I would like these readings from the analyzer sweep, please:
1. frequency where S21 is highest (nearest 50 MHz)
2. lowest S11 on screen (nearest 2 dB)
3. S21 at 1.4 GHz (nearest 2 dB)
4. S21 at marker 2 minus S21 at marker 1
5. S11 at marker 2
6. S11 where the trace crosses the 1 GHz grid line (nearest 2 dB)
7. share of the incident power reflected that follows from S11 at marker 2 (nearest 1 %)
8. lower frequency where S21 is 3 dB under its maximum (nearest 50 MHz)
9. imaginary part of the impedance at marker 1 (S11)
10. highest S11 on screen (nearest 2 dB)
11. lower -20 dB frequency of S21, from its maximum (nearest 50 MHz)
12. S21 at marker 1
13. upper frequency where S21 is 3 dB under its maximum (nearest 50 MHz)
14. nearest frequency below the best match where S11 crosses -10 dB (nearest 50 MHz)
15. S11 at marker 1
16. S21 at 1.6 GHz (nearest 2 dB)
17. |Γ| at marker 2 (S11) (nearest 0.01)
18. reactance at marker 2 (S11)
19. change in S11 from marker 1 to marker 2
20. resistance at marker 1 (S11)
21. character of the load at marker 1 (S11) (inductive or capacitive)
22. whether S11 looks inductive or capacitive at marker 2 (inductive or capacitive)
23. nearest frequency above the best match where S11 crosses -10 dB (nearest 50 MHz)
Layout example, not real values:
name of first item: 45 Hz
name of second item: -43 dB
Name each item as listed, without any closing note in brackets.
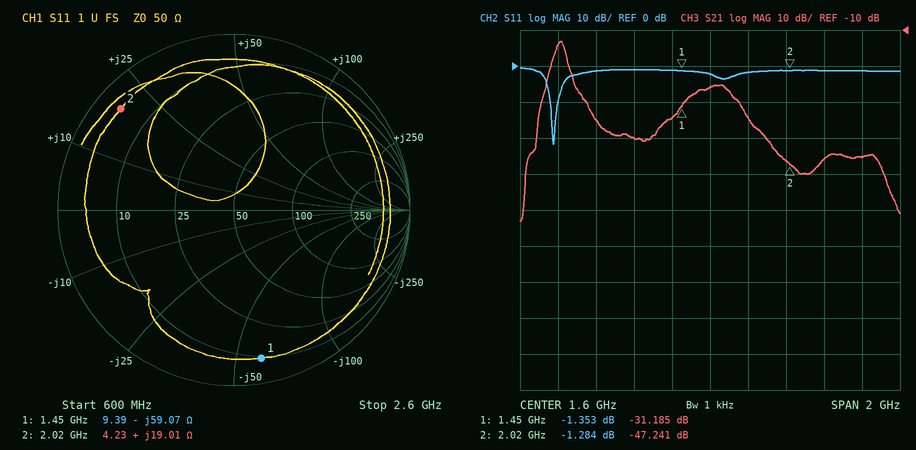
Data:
frequency where S21 is highest: 800 MHz
lowest S11 on screen: -22 dB
S21 at 1.4 GHz: -34 dB
S21 at marker 2 minus S21 at marker 1: -16.056 dB
S11 at marker 2: -1.284 dB
S11 where the trace crosses the 1 GHz grid line: -2 dB
share of the incident power reflected that follows from S11 at marker 2: 74 %
lower frequency where S21 is 3 dB under its maximum: 800 MHz
imaginary part of the impedance at marker 1: -59.07 Ω
highest S11 on screen: 0 dB
lower -20 dB frequency of S21, from its maximum: 700 MHz
S21 at marker 1: -31.185 dB
upper frequency where S21 is 3 dB under its maximum: 850 MHz
nearest frequency below the best match where S11 crosses -10 dB: 750 MHz
S11 at marker 1: -1.353 dB
S21 at 1.6 GHz: -26 dB
|Γ| at marker 2 (S11): 0.86
reactance at marker 2: +19.01 Ω
change in S11 from marker 1 to marker 2: 0.069 dB
resistance at marker 1: 9.39 Ω
character of the load at marker 1 (S11): capacitive
whether S11 looks inductive or capacitive at marker 2: inductive
nearest frequency above the best match where S11 crosses -10 dB: 800 MHz
